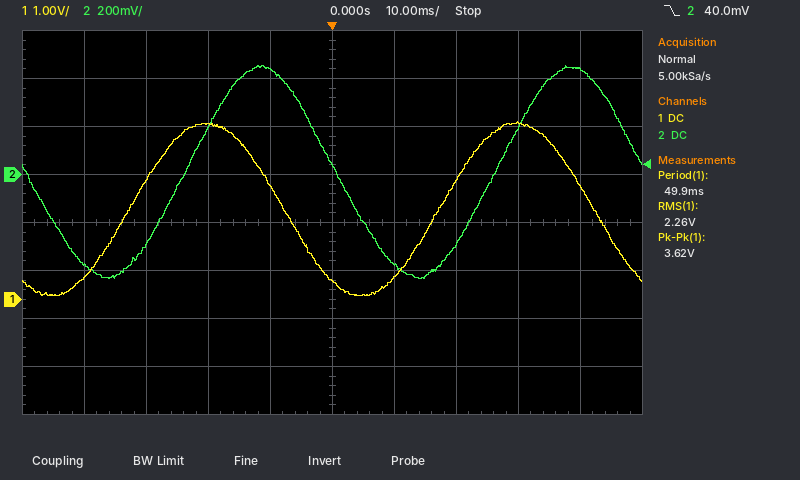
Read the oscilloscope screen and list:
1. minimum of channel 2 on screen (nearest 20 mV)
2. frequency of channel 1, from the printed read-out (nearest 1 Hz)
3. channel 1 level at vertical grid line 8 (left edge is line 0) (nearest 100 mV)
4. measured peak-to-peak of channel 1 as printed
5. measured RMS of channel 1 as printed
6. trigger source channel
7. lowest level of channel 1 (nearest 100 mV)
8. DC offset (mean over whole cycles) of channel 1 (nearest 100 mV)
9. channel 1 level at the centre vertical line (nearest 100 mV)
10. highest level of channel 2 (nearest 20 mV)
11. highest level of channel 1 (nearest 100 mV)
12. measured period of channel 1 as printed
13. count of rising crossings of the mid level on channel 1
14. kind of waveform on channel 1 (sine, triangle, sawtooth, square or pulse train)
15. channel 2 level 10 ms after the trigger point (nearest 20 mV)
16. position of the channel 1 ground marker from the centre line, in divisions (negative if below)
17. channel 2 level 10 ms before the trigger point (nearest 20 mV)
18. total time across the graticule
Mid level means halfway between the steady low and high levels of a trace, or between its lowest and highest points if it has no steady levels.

-440 mV
20 Hz
3.7 V
3.62 V
2.26 V
channel 2
100 mV
1.9 V
400 mV
460 mV
3.7 V
49.9 ms
2
sine
-380 mV
-1.6 div
440 mV
100 ms
